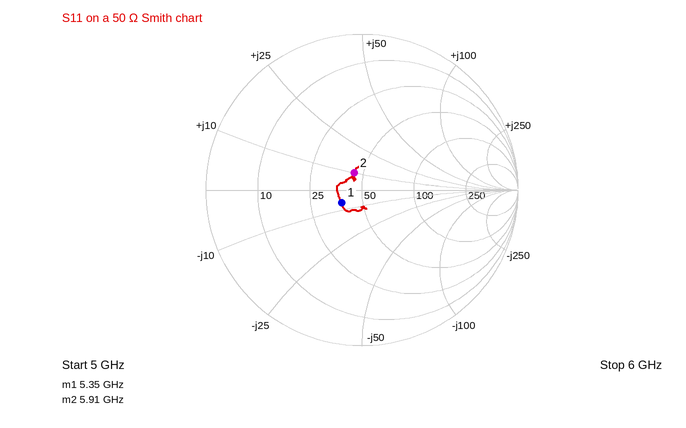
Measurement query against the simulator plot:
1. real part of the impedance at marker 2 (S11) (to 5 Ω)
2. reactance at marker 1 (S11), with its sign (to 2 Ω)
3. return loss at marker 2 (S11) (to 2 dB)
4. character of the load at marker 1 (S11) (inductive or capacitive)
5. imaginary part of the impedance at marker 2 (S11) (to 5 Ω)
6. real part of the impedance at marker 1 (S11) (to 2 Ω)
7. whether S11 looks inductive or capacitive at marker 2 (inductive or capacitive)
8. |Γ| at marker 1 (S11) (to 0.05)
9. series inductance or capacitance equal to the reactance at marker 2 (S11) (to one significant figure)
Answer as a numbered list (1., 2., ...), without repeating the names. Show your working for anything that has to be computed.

1. 45 Ω
2. -6 Ω
3. 18 dB
4. capacitive
5. +10 Ω
6. 38 Ω
7. inductive
8. 0.15
9. L = 10 Ω/(2π × 5.91 GHz) ≈ 269 pH, so 300 pH to one significant figure
